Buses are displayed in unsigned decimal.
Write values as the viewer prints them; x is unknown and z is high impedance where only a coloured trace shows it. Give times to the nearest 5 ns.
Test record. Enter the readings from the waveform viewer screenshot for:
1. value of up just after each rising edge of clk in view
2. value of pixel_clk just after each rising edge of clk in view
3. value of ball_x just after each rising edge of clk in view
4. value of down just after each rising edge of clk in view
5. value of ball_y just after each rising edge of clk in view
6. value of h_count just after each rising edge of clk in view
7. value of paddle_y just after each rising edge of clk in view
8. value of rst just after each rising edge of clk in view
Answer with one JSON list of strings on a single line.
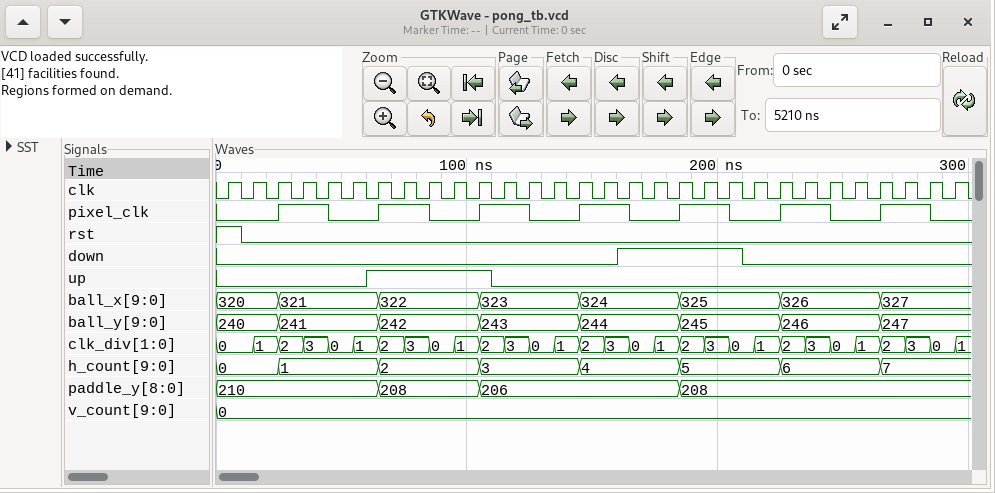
["0 0 0 0 0 0 1 1 1 1 1 0 0 0 0 0 0 0 0 0 0 0 0 0 0 0 0 0 0 0", "0 0 1 1 0 0 1 1 0 0 1 1 0 0 1 1 0 0 1 1 0 0 1 1 0 0 1 1 0 0", "320, 320, 321, 321, 321, 321, 322, 322, 322, 322, 323, 323, 323, 323, 324, 324, 324, 324, 325, 325, 325, 325, 326, 326, 326, 326, 327, 327, 327, 327", "0 0 0 0 0 0 0 0 0 0 0 0 0 0 0 0 1 1 1 1 1 0 0 0 0 0 0 0 0 0", "240, 240, 241, 241, 241, 241, 242, 242, 242, 242, 243, 243, 243, 243, 244, 244, 244, 244, 245, 245, 245, 245, 246, 246, 246, 246, 247, 247, 247, 247", "0, 0, 1, 1, 1, 1, 2, 2, 2, 2, 3, 3, 3, 3, 4, 4, 4, 4, 5, 5, 5, 5, 6, 6, 6, 6, 7, 7, 7, 7", "210, 210, 210, 210, 210, 210, 208, 208, 208, 208, 206, 206, 206, 206, 206, 206, 206, 206, 208, 208, 208, 208, 208, 208, 208, 208, 208, 208, 208, 208", "1 0 0 0 0 0 0 0 0 0 0 0 0 0 0 0 0 0 0 0 0 0 0 0 0 0 0 0 0 0"]
